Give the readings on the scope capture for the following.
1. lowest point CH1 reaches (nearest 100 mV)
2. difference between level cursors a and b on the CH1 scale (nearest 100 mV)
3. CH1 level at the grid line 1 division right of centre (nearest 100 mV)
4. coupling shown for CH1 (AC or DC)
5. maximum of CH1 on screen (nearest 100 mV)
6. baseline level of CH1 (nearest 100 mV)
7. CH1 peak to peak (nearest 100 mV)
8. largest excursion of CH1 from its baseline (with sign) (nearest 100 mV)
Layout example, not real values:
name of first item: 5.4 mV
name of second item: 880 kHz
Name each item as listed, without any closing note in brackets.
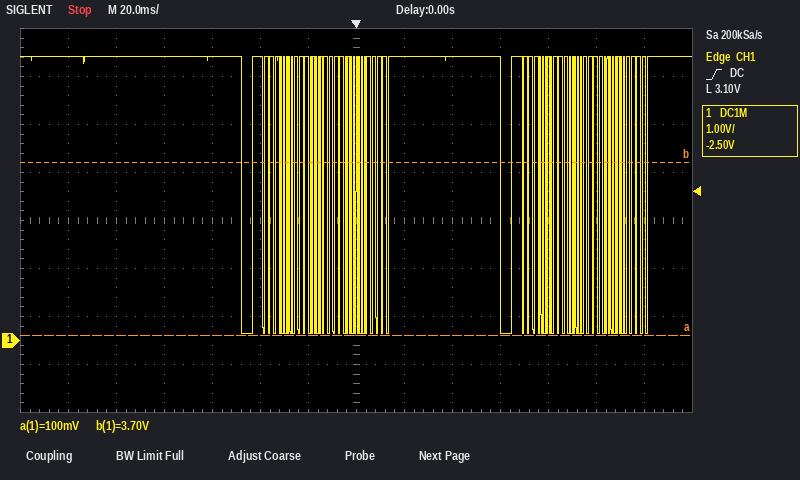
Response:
lowest point CH1 reaches: 100 mV
difference between level cursors a and b on the CH1 scale: 3.6 V
CH1 level at the grid line 1 division right of centre: 5.9 V
coupling shown for CH1: DC
maximum of CH1 on screen: 5.9 V
baseline level of CH1: 5.9 V
CH1 peak to peak: 5.8 V
largest excursion of CH1 from its baseline (with sign): -5.8 V
